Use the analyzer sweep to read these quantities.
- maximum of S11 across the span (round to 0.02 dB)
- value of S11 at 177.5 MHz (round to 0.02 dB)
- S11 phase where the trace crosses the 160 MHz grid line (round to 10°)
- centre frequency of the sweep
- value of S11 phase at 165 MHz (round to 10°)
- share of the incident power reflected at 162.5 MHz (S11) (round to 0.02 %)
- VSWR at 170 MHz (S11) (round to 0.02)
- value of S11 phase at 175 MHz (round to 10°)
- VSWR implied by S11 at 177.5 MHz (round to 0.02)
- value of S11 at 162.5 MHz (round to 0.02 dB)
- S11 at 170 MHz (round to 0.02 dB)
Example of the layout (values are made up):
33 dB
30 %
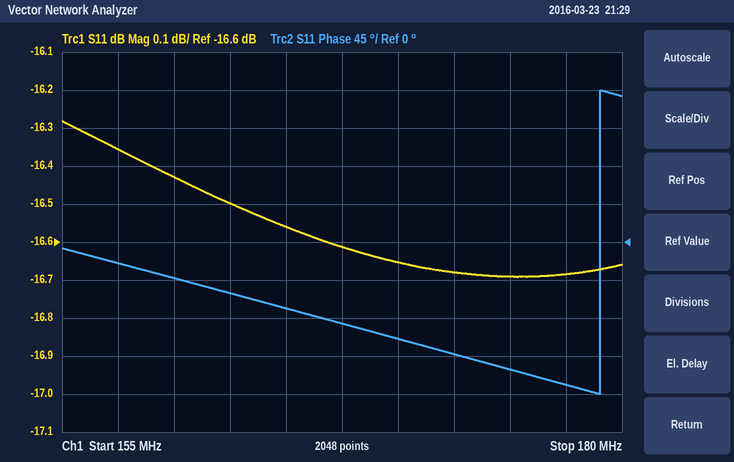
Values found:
-16.28 dB
-16.68 dB
-40°
167.5 MHz
-80°
2.24 %
1.34
-150°
1.34
-16.50 dB
-16.66 dB
